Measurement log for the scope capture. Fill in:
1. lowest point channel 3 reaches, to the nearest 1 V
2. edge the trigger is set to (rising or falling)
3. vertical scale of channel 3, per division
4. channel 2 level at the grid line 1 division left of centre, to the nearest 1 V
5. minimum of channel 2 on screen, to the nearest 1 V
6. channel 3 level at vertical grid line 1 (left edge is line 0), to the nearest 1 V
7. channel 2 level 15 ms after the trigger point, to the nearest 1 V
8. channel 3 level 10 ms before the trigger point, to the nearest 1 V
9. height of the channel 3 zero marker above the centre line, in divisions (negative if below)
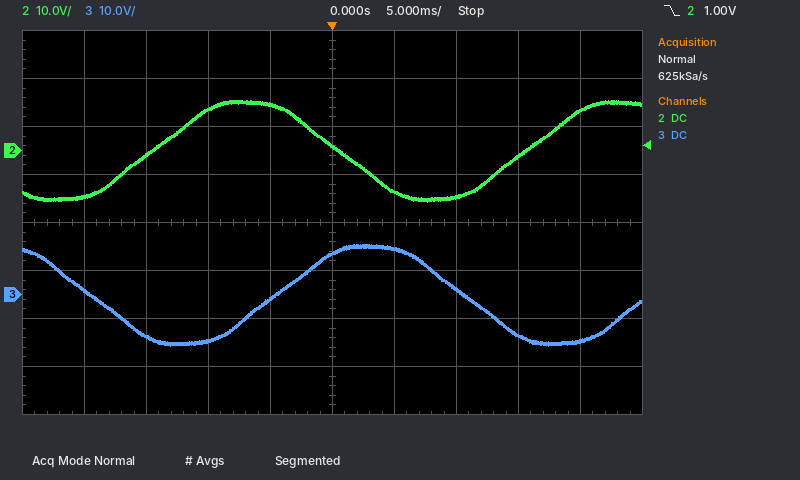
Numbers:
-11 V
falling
10 V
10 V
-11 V
1 V
-1 V
-10 V
-1.5 div
